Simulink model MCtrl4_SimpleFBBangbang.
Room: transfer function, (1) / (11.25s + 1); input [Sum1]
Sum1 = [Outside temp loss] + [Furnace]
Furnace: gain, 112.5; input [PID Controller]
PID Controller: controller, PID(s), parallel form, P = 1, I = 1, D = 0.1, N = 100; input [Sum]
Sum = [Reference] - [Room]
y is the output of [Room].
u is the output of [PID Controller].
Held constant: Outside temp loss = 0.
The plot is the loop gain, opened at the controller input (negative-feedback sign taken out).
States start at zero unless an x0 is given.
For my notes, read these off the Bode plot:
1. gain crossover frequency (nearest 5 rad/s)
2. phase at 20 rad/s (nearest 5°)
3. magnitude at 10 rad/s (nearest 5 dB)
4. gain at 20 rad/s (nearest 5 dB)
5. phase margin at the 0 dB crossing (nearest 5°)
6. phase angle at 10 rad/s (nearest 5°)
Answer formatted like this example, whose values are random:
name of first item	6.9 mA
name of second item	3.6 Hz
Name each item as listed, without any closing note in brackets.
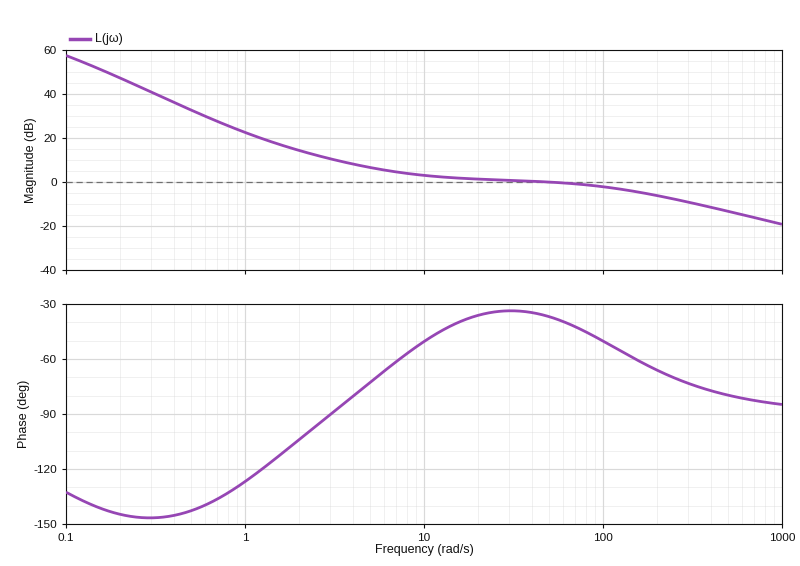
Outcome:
gain crossover frequency	50 rad/s
phase at 20 rad/s	-35°
magnitude at 10 rad/s	5 dB
gain at 20 rad/s	0 dB
phase margin at the 0 dB crossing	145°
phase angle at 10 rad/s	-50°
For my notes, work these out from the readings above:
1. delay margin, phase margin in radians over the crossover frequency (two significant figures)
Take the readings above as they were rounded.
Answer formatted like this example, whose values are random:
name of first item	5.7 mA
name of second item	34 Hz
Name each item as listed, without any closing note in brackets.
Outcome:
delay margin, phase margin in radians over the crossover frequency	0.051 s
